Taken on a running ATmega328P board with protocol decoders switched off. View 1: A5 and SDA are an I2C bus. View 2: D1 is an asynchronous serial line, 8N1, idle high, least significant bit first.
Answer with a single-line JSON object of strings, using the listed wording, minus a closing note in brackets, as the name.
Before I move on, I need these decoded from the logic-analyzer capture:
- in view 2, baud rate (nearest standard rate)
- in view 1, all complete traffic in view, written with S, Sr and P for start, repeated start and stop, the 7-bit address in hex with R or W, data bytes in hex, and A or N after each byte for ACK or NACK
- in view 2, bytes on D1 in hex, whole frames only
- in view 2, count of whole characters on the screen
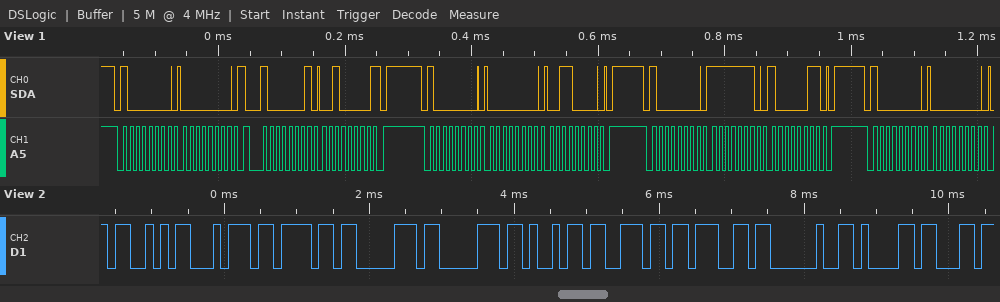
{"in view 2, baud rate": "9600 baud", "in view 1, all complete traffic in view, written with S, Sr and P for start, repeated start and stop, the 7-bit address in hex with R or W, data bytes in hex, and A or N after each byte for ACK or NACK": "S 40W A 00 A Sr 40R A 20 N P S 40W A 00 A 30 A P S 40W A FE A 83 A P S 40W A 00 A", "in view 2, bytes on D1 in hex, whole frames only": "53 74 6F 70 70 69 6E 67 20 61", "in view 2, count of whole characters on the screen": "10"}
